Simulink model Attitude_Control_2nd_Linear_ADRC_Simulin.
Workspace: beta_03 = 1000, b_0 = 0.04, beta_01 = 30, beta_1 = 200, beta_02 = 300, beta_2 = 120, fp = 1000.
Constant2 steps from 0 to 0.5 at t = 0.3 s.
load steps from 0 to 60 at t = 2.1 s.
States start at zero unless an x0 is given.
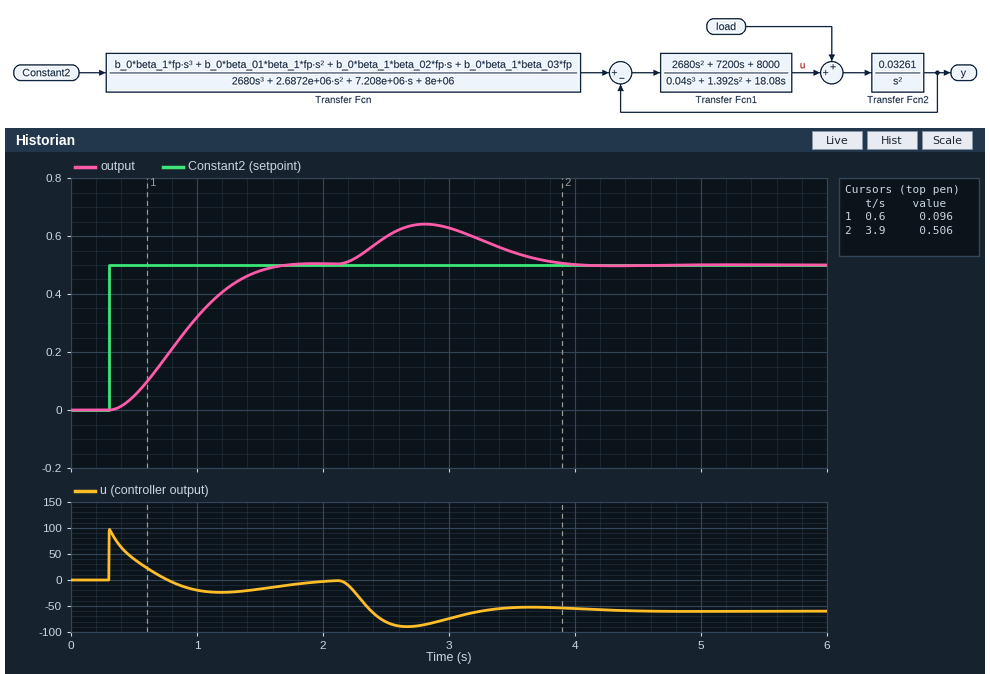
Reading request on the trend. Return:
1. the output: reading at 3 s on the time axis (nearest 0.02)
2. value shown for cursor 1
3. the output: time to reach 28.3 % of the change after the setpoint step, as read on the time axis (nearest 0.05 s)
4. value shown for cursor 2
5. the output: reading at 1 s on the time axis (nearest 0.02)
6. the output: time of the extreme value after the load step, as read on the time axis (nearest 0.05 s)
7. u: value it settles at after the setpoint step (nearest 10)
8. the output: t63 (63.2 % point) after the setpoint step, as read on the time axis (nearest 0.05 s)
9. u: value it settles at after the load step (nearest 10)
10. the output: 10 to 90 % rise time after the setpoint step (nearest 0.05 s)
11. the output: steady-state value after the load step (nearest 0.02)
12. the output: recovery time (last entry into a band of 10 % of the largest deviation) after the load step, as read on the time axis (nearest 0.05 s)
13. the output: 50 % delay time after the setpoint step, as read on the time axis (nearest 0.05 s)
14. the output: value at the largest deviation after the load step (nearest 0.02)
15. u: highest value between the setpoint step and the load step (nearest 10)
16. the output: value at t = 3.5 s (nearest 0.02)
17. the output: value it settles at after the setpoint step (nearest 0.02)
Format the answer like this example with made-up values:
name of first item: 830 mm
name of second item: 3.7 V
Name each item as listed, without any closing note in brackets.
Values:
the output: reading at 3 s on the time axis: 0.62
value shown for cursor 1: 0.096
the output: time to reach 28.3 % of the change after the setpoint step, as read on the time axis: 0.70 s
value shown for cursor 2: 0.506
the output: reading at 1 s on the time axis: 0.32
the output: time of the extreme value after the load step, as read on the time axis: 2.80 s
u: value it settles at after the setpoint step: 0
the output: t63 (63.2 % point) after the setpoint step, as read on the time axis: 1.00 s
u: value it settles at after the load step: -60
the output: 10 to 90 % rise time after the setpoint step: 0.85 s
the output: steady-state value after the load step: 0.50
the output: recovery time (last entry into a band of 10 % of the largest deviation) after the load step, as read on the time axis: 3.80 s
the output: 50 % delay time after the setpoint step, as read on the time axis: 0.85 s
the output: value at the largest deviation after the load step: 0.64
u: highest value between the setpoint step and the load step: 100
the output: value at t = 3.5 s: 0.54
the output: value it settles at after the setpoint step: 0.50
